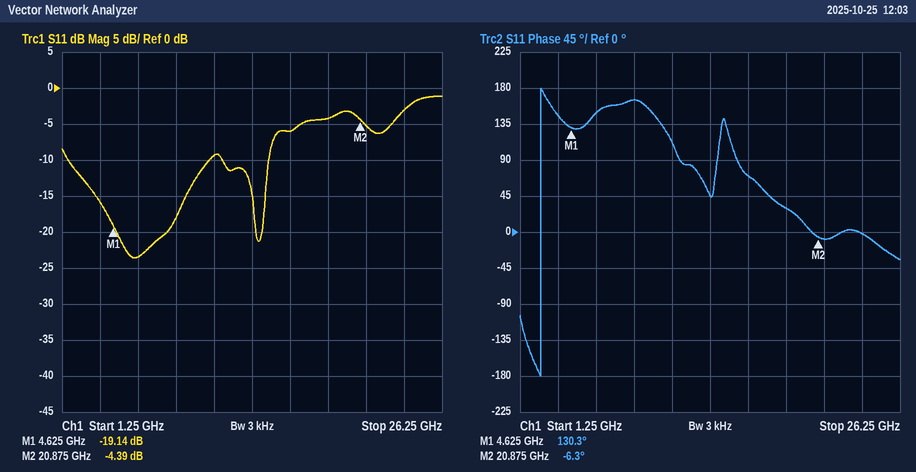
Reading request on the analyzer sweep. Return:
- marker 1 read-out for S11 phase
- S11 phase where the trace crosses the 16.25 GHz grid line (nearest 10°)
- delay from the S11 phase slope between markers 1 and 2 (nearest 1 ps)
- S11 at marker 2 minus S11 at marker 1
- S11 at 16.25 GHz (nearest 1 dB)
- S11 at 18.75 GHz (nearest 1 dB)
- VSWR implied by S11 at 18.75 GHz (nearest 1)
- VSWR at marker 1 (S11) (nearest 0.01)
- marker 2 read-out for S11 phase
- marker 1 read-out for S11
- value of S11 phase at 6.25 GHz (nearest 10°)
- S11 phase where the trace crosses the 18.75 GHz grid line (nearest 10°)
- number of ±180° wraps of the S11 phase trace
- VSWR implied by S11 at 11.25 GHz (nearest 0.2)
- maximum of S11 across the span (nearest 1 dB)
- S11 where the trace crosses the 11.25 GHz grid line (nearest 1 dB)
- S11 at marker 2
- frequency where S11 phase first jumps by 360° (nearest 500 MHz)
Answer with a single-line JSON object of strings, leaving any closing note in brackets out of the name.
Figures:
{"marker 1 read-out for S11 phase": "130.3°", "S11 phase where the trace crosses the 16.25 GHz grid line": "70°", "delay from the S11 phase slope between markers 1 and 2": "23 ps", "S11 at marker 2 minus S11 at marker 1": "14.75 dB", "S11 at 16.25 GHz": "-6 dB", "S11 at 18.75 GHz": "-4 dB", "VSWR implied by S11 at 18.75 GHz": "4", "VSWR at marker 1 (S11)": "1.25", "marker 2 read-out for S11 phase": "-6.3°", "marker 1 read-out for S11": "-19.14 dB", "value of S11 phase at 6.25 GHz": "150°", "S11 phase where the trace crosses the 18.75 GHz grid line": "30°", "number of ±180° wraps of the S11 phase trace": "1", "VSWR implied by S11 at 11.25 GHz": "2.0", "maximum of S11 across the span": "-1 dB", "S11 where the trace crosses the 11.25 GHz grid line": "-9 dB", "S11 at marker 2": "-4.39 dB", "frequency where S11 phase first jumps by 360°": "2.5 GHz"}
